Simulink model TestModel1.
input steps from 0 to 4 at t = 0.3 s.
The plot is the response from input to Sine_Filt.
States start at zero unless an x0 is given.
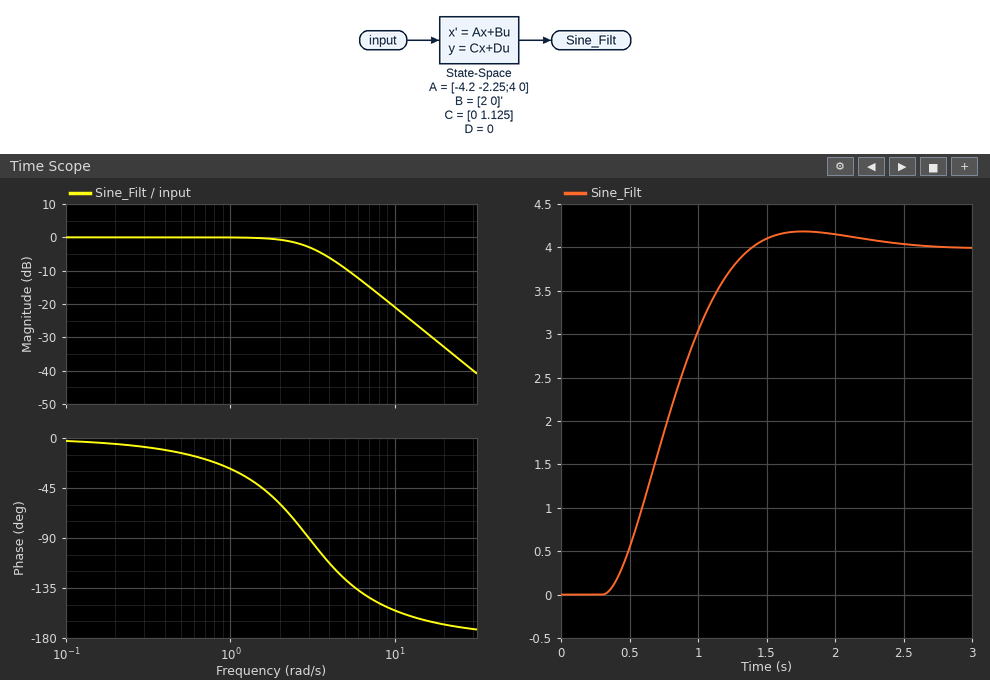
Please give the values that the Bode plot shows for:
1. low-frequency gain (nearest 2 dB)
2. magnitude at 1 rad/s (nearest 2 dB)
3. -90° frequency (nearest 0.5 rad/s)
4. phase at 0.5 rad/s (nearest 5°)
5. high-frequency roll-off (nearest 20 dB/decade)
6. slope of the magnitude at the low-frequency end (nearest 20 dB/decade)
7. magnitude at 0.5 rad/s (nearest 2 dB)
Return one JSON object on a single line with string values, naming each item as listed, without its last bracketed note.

{"low-frequency gain": "0 dB", "magnitude at 1 rad/s": "0 dB", "-90° frequency": "3.0 rad/s", "phase at 0.5 rad/s": "-15°", "high-frequency roll-off": "-40 dB/decade", "slope of the magnitude at the low-frequency end": "0 dB/decade", "magnitude at 0.5 rad/s": "0 dB"}
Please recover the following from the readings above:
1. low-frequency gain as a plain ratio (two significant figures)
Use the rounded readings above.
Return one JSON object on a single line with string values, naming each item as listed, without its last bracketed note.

{"low-frequency gain as a plain ratio": "1.0"}
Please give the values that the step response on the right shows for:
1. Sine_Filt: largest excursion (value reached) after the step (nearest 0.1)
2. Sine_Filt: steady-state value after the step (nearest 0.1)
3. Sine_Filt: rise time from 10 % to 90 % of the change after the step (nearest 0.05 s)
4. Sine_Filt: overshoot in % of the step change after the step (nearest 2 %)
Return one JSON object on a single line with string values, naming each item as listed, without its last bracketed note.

{"Sine_Filt: largest excursion (value reached) after the step": "4.2", "Sine_Filt: steady-state value after the step": "4.0", "Sine_Filt: rise time from 10 % to 90 % of the change after the step": "0.70 s", "Sine_Filt: overshoot in % of the step change after the step": "4 %"}
